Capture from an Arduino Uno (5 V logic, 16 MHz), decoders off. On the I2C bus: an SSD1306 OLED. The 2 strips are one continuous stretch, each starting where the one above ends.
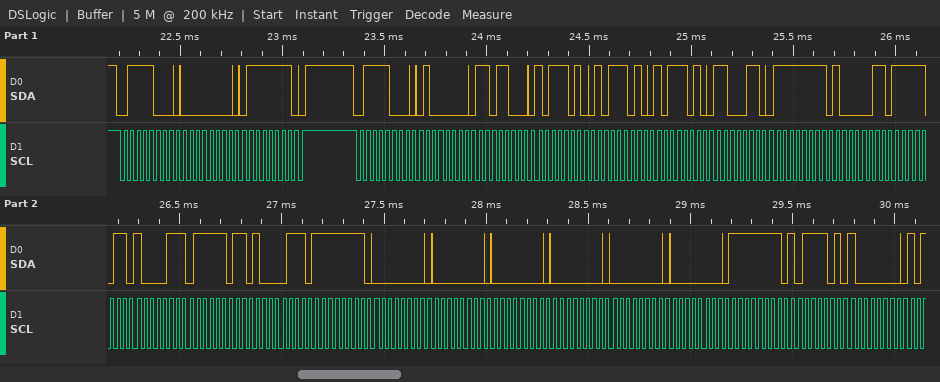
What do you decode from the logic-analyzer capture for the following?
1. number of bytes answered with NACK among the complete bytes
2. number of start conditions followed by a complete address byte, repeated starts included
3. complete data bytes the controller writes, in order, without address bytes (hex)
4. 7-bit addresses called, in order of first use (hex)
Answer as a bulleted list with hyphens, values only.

- 0
- 2
- 00 7F 40 D8 BA BA BA C6 FF 83 FB 87 FB 87 FF 00 00 00 00 00 00 FF BD 80
- 0x3C
